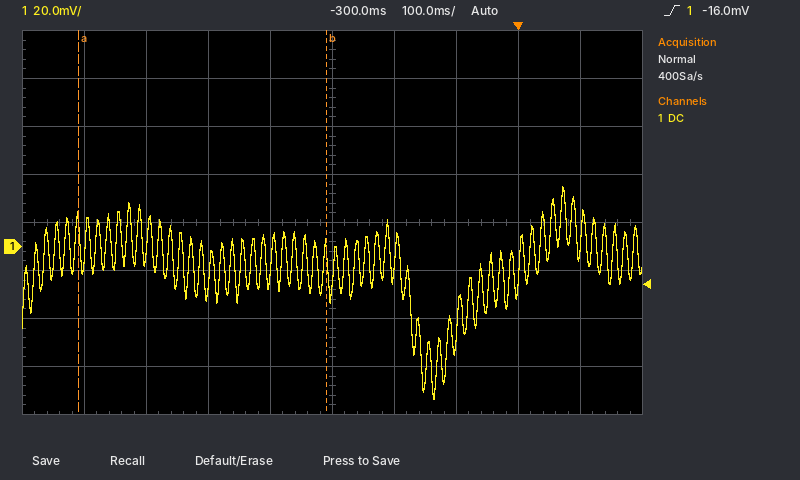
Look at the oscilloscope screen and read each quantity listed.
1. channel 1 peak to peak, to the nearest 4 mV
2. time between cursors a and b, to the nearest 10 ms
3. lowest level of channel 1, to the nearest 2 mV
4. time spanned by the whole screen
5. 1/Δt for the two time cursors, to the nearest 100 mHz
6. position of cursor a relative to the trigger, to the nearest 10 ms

88 mV
400 ms
-64 mV
1 s
2.5 Hz
-710 ms
